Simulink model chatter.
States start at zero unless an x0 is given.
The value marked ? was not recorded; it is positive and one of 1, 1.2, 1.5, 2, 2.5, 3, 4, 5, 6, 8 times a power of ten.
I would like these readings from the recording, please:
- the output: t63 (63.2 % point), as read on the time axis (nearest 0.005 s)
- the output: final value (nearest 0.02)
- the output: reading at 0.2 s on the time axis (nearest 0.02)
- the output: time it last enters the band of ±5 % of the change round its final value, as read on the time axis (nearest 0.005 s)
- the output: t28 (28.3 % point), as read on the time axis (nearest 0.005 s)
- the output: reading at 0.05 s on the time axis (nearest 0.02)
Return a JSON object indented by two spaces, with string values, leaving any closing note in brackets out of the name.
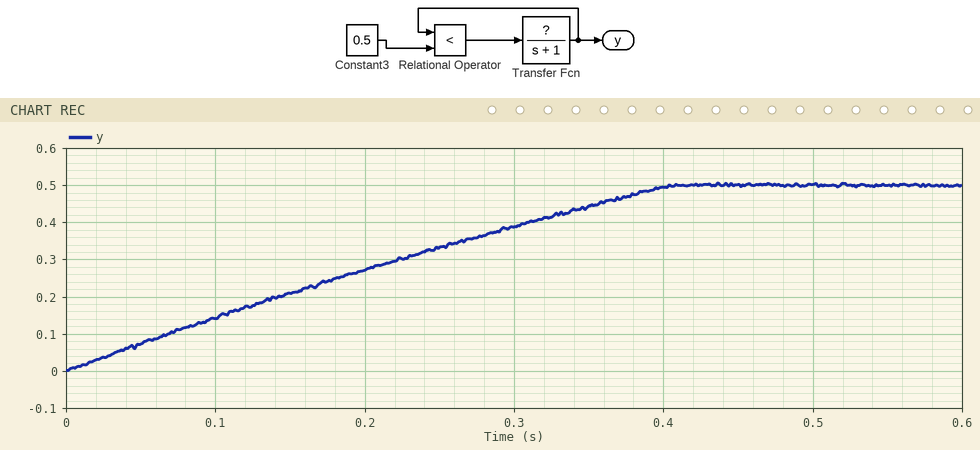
{
  "the output: t63 (63.2 % point), as read on the time axis": "0.235 s",
  "the output: final value": "0.50",
  "the output: reading at 0.2 s on the time axis": "0.28",
  "the output: time it last enters the band of ±5 % of the change round its final value, as read on the time axis": "0.380 s",
  "the output: t28 (28.3 % point), as read on the time axis": "0.100 s",
  "the output: reading at 0.05 s on the time axis": "0.08"
}
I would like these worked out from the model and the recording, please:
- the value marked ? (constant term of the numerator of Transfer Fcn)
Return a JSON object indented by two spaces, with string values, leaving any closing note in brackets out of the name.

{
  "the value marked ?": "1.5"
}
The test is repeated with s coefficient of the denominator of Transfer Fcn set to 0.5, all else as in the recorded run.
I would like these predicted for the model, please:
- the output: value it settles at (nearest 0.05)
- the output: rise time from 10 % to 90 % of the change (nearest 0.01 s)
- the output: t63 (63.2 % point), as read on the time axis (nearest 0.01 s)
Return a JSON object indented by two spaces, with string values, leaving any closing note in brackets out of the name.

{
  "the output: value it settles at": "0.50",
  "the output: rise time from 10 % to 90 % of the change": "0.16 s",
  "the output: t63 (63.2 % point), as read on the time axis": "0.12 s"
}
